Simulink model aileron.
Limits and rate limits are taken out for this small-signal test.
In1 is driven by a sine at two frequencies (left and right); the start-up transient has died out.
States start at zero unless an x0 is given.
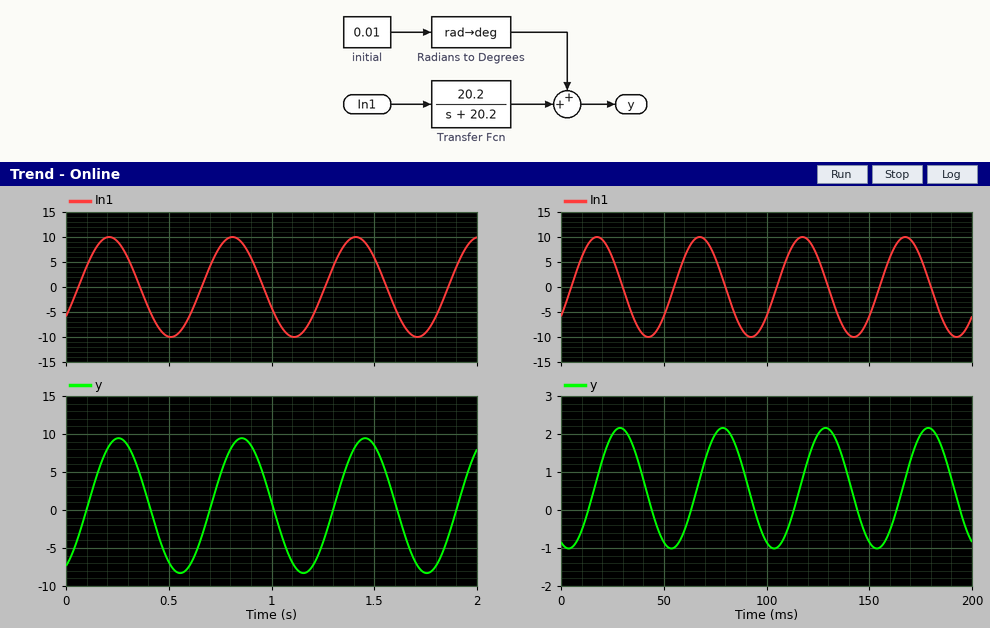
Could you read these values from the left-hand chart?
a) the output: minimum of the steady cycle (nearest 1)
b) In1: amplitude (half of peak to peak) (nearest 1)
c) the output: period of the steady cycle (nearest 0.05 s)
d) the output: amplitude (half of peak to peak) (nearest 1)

-8
10
0.60 s
9
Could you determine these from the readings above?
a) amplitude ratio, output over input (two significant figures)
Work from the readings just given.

0.90
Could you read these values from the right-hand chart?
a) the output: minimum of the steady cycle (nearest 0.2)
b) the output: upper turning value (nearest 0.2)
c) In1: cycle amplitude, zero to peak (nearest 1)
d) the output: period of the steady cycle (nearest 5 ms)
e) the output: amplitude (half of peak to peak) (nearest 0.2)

-1.0
2.2
10
50 ms
1.6
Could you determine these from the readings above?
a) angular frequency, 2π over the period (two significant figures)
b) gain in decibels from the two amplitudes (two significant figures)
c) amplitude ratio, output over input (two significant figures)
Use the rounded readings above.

0.13 rad/ms
-16 dB
0.16
